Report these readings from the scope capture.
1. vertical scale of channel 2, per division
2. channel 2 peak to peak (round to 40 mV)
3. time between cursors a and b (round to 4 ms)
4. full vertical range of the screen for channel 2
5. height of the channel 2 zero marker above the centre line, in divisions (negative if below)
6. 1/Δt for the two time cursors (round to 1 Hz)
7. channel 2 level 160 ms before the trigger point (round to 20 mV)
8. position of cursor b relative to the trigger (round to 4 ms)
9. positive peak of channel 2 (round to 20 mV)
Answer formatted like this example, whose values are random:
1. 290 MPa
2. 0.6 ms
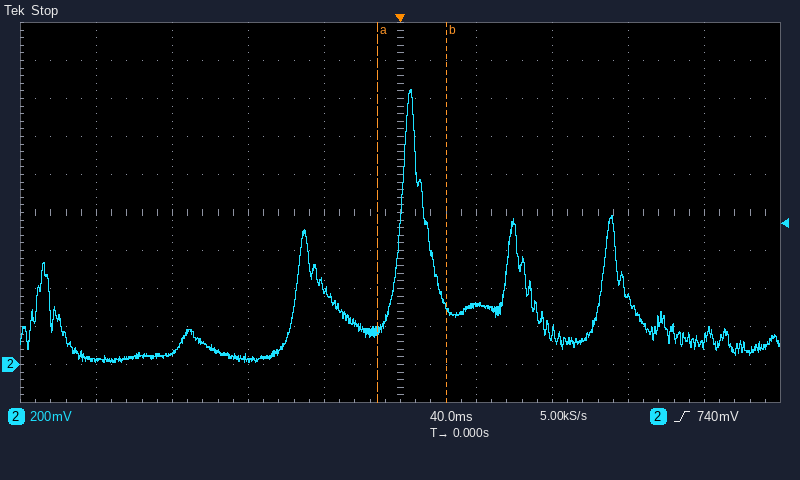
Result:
1. 200 mV
2. 1.44 V
3. 36 ms
4. 2 V
5. -4.0 div
6. 28 Hz
7. 20 mV
8. +24 ms
9. 1.44 V
